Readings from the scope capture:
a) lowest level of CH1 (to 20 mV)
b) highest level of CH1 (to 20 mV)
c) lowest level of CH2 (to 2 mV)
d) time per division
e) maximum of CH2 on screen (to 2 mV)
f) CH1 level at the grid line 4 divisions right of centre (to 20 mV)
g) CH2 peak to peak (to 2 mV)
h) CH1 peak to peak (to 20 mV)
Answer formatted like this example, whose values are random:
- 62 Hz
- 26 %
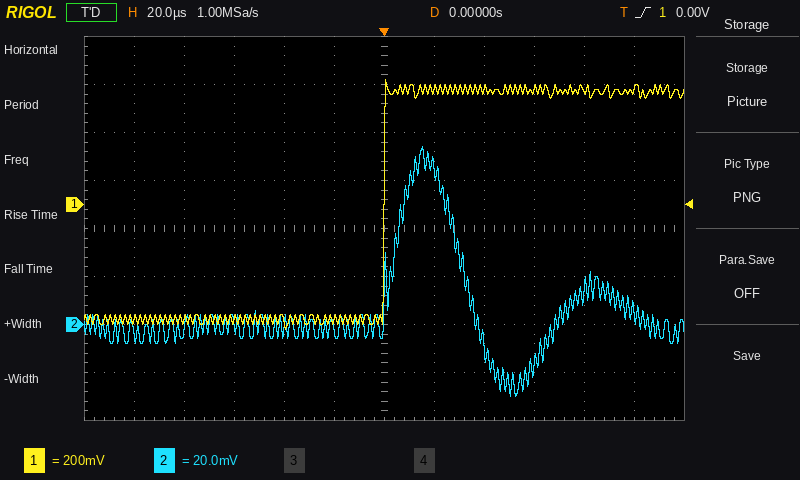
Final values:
- -520 mV
- 520 mV
- -30 mV
- 20 µs
- 74 mV
- 480 mV
- 104 mV
- 1.04 V
